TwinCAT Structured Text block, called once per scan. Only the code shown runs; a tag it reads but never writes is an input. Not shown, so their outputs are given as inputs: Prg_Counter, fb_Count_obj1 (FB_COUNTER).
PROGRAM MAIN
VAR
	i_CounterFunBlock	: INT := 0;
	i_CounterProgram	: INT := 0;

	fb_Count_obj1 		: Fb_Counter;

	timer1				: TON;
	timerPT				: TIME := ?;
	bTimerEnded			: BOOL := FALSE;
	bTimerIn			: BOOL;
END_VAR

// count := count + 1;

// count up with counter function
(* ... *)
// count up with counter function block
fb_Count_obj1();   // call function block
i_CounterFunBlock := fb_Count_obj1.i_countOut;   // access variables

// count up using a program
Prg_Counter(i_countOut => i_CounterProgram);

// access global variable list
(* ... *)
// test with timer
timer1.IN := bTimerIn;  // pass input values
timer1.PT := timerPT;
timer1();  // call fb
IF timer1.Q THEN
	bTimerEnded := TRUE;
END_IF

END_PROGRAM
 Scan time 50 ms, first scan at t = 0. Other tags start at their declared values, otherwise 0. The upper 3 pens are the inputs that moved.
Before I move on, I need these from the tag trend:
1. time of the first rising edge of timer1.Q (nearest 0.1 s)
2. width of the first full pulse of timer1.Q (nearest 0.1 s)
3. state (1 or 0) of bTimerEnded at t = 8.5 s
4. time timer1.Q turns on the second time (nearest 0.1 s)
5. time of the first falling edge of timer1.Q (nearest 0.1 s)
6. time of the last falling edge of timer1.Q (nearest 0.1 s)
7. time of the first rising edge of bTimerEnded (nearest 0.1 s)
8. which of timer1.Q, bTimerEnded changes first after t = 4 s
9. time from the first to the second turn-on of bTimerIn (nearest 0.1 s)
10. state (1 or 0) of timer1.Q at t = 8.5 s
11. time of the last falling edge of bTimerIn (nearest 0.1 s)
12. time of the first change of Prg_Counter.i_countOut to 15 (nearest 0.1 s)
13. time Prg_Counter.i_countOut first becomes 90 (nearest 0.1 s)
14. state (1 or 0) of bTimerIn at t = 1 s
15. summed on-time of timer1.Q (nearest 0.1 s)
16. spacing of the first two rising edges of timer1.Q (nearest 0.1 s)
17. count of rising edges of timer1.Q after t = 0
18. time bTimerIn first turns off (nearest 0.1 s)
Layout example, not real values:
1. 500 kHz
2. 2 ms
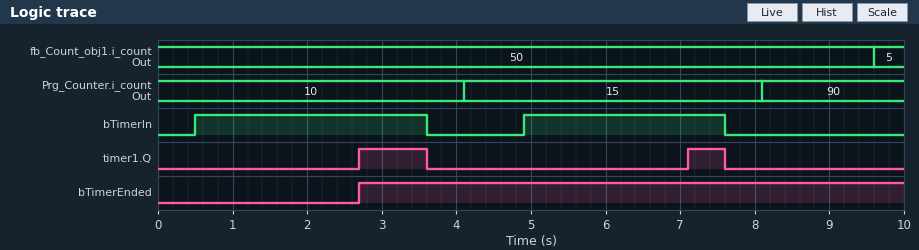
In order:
1. 2.7 s
2. 0.9 s
3. 1
4. 7.1 s
5. 3.6 s
6. 7.6 s
7. 2.7 s
8. timer1.Q
9. 4.4 s
10. 0
11. 7.6 s
12. 4.1 s
13. 8.1 s
14. 1
15. 1.4 s
16. 4.4 s
17. 2
18. 3.6 s
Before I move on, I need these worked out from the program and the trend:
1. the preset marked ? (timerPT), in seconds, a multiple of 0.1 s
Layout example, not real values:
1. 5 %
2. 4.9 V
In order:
1. 2.2 s
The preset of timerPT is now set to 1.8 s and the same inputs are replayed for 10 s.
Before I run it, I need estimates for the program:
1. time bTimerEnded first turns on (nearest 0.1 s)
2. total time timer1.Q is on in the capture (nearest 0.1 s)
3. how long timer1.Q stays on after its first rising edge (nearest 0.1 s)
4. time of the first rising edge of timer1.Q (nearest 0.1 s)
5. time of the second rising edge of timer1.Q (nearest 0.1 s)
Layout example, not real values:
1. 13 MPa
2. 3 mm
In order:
1. 2.3 s
2. 2.2 s
3. 1.3 s
4. 2.3 s
5. 6.7 s
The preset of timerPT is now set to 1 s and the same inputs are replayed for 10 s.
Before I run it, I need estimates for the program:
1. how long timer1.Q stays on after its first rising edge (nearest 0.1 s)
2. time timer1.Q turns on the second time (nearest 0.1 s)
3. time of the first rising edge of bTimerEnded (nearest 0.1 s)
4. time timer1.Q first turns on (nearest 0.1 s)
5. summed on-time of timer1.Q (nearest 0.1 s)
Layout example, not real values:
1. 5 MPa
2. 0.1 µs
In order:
1. 2.1 s
2. 5.9 s
3. 1.5 s
4. 1.5 s
5. 3.8 s
